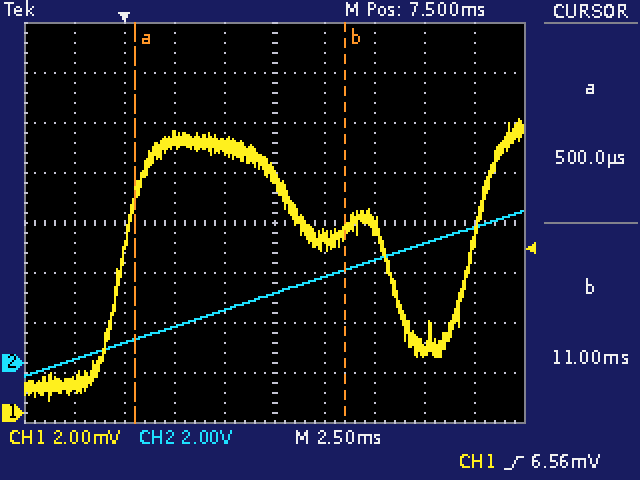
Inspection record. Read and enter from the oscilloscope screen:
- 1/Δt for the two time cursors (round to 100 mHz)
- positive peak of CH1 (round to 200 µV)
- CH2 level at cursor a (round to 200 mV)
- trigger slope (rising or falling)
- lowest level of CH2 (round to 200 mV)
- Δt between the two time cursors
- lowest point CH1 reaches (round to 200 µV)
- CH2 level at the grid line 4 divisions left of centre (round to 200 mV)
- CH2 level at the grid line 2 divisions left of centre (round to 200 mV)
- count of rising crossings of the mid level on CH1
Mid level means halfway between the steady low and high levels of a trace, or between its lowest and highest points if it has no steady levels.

95.2 Hz
11.8 mV
1.0 V
rising
-600 mV
10.50 ms
400 µV
200 mV
1.4 V
2
